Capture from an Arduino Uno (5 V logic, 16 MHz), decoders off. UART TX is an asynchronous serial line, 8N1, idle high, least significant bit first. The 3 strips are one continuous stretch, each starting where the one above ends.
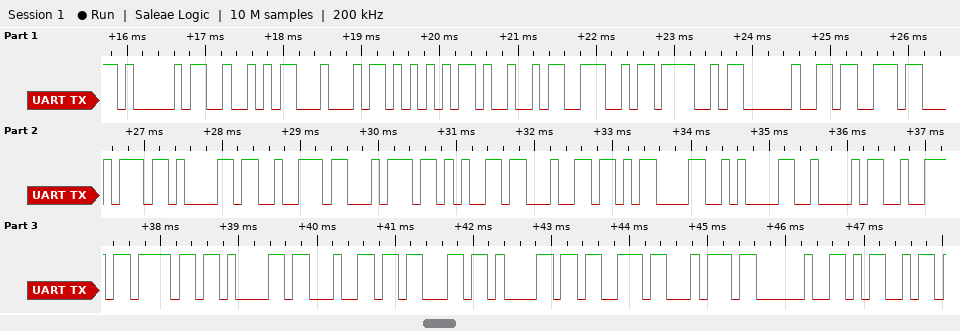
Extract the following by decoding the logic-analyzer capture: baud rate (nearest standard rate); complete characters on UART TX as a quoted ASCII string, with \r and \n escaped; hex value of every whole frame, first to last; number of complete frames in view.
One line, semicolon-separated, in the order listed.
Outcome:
9600 baud; "ARDUINO started\r\nBroadcast M"; 41 52 44 55 49 4E 4F 20 73 74 61 72 74 65 64 0D 0A 42 72 6F 61 64 63 61 73 74 20 4D; 28
